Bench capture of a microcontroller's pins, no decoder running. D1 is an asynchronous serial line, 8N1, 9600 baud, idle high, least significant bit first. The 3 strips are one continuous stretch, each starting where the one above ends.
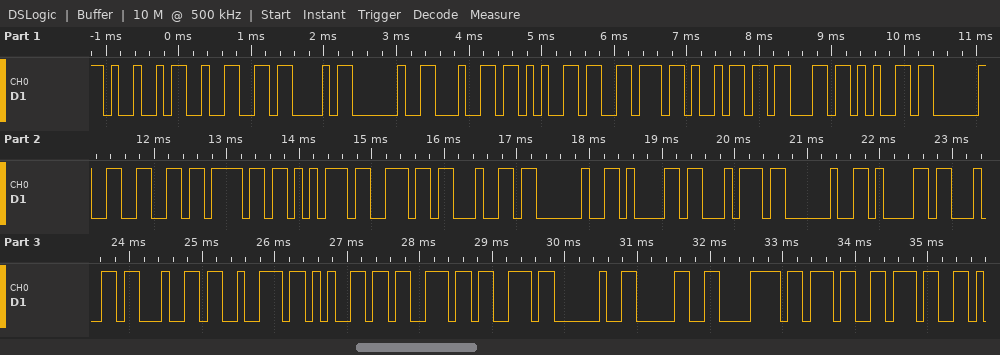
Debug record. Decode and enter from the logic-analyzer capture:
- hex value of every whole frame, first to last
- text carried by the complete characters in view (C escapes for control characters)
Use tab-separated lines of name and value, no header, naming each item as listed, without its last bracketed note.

hex value of every whole frame, first to last	0x49 0x32 0x43 0x20 0x64 0x65 0x76 0x69 0x63 0x65 0x20 0x66 0x6F 0x75 0x6E 0x64 0x20 0x61 0x74 0x20 0x61 0x64 0x64 0x72 0x65 0x73 0x73 0x20 0x30 0x78 0x37 0x37
text carried by the complete characters in view	"I2C device found at address 0x77"
